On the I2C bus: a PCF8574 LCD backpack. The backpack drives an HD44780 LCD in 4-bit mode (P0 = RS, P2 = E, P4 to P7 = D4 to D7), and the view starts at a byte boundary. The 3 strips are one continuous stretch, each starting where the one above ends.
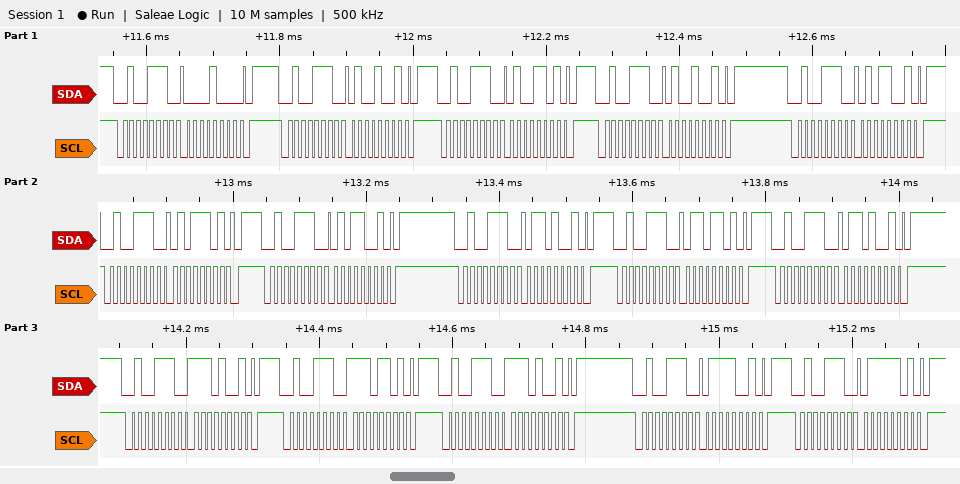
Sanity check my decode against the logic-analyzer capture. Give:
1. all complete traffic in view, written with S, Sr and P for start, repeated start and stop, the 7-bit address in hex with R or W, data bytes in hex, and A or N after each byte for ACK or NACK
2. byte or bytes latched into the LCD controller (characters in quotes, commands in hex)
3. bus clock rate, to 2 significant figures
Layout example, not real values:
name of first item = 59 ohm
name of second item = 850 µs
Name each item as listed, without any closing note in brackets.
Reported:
all complete traffic in view, written with S, Sr and P for start, repeated start and stop, the 7-bit address in hex with R or W, data bytes in hex, and A or N after each byte for ACK or NACK = S 27W A 08 A P S 27W A 49 A P S 27W A 4D A P S 27W A 49 A P S 27W A 59 A P S 27W A 5D A P S 27W A 59 A P S 27W A 69 A P S 27W A 6D A P S 27W A 69 A P S 27W A E9 A P S 27W A ED A P S 27W A E9 A P S 27W A 79 A P S 27W A 7D A P
byte or bytes latched into the LCD controller = 'E' 'n'
bus clock rate, to 2 significant figures = 100 kHz
